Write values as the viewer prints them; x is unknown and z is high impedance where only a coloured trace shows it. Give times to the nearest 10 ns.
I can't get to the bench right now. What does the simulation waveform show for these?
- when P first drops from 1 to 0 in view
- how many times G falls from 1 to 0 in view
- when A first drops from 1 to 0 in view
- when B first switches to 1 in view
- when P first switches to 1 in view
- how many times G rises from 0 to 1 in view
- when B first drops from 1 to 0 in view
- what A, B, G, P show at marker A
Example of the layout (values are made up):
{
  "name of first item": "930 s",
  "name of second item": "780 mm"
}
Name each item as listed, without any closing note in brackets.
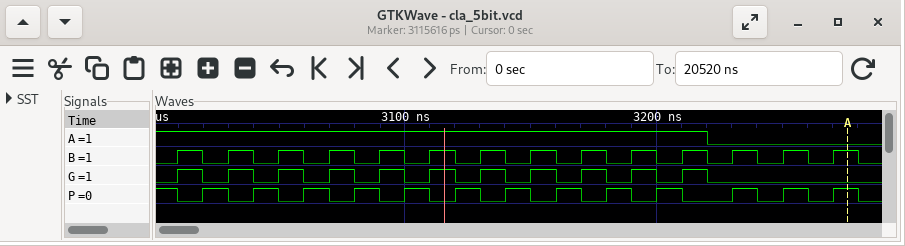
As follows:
{
  "when P first drops from 1 to 0 in view": "3010 ns",
  "how many times G falls from 1 to 0 in view": "11",
  "when A first drops from 1 to 0 in view": "3220 ns",
  "when B first switches to 1 in view": "3010 ns",
  "when P first switches to 1 in view": "3020 ns",
  "how many times G rises from 0 to 1 in view": "11",
  "when B first drops from 1 to 0 in view": "3020 ns",
  "what A, B, G, P show at marker A": "A=0, B=1, G=0, P=1"
}
